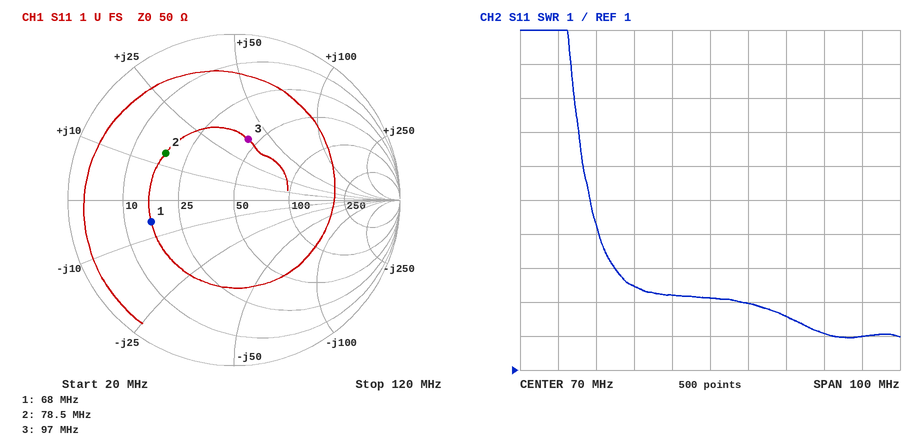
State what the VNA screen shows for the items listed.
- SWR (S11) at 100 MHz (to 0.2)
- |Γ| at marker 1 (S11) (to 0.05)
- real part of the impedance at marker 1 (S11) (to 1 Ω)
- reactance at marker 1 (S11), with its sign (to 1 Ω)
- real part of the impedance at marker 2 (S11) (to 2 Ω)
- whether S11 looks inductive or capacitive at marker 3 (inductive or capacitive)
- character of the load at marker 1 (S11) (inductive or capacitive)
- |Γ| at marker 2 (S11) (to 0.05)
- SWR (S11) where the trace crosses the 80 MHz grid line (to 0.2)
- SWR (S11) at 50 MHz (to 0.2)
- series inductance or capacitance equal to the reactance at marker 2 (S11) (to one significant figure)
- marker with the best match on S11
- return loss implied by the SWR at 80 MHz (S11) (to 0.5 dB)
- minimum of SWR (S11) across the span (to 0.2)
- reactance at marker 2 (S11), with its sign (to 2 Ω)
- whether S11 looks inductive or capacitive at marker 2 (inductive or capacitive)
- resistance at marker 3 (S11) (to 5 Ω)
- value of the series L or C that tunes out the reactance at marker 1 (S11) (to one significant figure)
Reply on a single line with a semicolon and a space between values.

2.0; 0.50; 16 Ω; -6 Ω; 18 Ω; inductive; capacitive; 0.50; 3.0; 3.4; 30 nH; marker 3; 6.0 dB; 2.0; +14 Ω; inductive; 45 Ω; 10 nH
